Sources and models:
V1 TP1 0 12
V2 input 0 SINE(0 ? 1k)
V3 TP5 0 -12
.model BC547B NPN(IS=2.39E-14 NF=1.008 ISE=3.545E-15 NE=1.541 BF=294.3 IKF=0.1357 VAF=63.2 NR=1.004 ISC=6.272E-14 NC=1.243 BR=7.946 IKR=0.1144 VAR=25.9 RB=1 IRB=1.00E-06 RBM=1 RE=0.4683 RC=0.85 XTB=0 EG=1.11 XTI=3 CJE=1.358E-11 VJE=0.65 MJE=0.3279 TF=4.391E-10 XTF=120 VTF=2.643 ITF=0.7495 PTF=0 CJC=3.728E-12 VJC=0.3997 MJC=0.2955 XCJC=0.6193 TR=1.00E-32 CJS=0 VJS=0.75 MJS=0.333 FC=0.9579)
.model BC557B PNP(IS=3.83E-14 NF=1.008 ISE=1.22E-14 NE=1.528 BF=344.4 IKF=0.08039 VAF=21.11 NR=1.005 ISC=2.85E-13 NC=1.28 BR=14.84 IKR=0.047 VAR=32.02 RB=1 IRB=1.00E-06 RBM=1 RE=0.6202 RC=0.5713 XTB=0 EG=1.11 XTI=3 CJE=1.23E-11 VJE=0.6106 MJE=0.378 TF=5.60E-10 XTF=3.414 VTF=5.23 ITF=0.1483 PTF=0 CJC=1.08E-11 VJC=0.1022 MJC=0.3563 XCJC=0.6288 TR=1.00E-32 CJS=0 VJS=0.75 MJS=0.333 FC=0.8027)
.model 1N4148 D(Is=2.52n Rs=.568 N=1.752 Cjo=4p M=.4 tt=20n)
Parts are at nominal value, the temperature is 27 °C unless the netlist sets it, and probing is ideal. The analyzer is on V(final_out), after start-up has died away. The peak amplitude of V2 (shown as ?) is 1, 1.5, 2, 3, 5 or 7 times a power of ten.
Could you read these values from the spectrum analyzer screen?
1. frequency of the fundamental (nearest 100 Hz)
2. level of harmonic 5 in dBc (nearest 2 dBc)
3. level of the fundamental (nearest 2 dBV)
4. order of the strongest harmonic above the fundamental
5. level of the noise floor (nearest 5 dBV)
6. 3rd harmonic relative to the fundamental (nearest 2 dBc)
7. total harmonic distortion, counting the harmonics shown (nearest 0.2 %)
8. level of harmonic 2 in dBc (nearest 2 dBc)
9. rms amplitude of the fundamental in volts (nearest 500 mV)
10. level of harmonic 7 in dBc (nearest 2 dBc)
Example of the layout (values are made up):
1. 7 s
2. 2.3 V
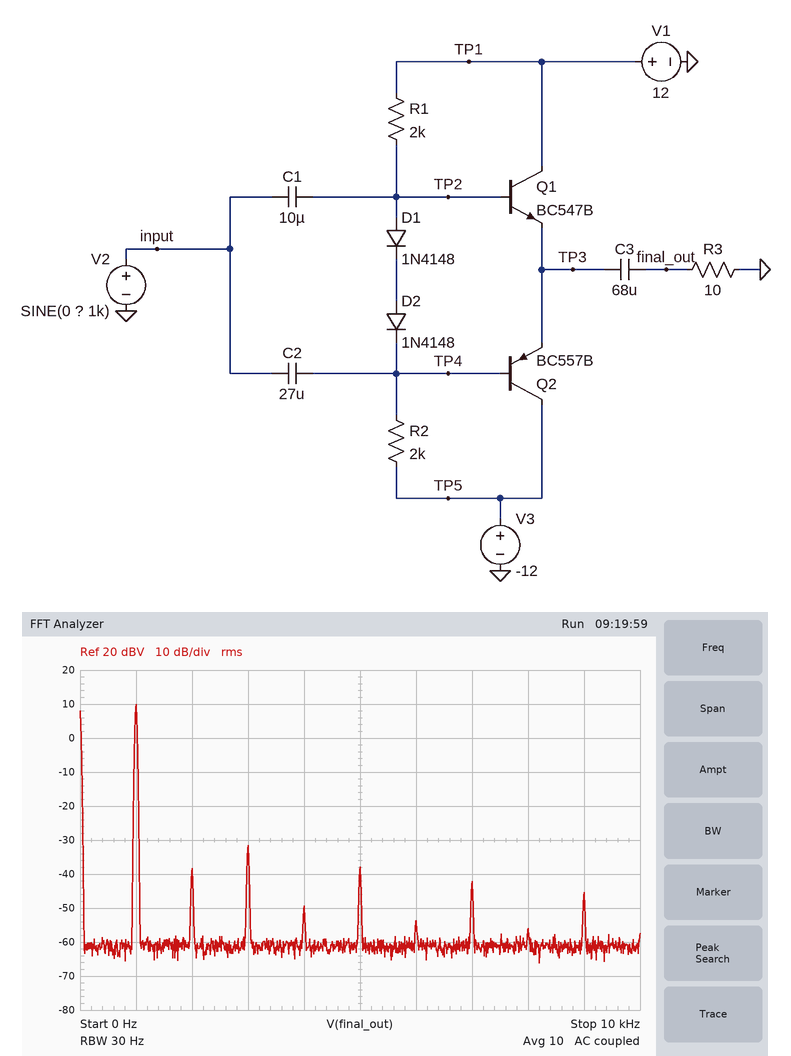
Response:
1. 1.0 kHz
2. -48 dBc
3. 10 dBV
4. 3
5. -60 dBV
6. -42 dBc
7. 1.0 %
8. -48 dBc
9. 3.0 V
10. -52 dBc
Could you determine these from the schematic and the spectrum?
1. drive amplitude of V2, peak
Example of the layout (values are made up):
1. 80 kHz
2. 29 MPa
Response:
1. 5 V
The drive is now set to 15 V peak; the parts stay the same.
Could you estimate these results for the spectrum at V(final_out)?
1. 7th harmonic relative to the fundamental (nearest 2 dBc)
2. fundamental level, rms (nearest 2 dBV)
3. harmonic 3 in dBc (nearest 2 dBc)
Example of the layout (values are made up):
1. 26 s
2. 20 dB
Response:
1. -28 dBc
2. 16 dBV
3. -16 dBc
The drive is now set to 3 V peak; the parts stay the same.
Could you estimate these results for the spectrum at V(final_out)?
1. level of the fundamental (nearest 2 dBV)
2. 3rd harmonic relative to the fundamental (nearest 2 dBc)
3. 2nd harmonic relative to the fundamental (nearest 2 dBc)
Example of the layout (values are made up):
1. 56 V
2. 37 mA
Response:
1. 6 dBV
2. -40 dBc
3. -50 dBc
